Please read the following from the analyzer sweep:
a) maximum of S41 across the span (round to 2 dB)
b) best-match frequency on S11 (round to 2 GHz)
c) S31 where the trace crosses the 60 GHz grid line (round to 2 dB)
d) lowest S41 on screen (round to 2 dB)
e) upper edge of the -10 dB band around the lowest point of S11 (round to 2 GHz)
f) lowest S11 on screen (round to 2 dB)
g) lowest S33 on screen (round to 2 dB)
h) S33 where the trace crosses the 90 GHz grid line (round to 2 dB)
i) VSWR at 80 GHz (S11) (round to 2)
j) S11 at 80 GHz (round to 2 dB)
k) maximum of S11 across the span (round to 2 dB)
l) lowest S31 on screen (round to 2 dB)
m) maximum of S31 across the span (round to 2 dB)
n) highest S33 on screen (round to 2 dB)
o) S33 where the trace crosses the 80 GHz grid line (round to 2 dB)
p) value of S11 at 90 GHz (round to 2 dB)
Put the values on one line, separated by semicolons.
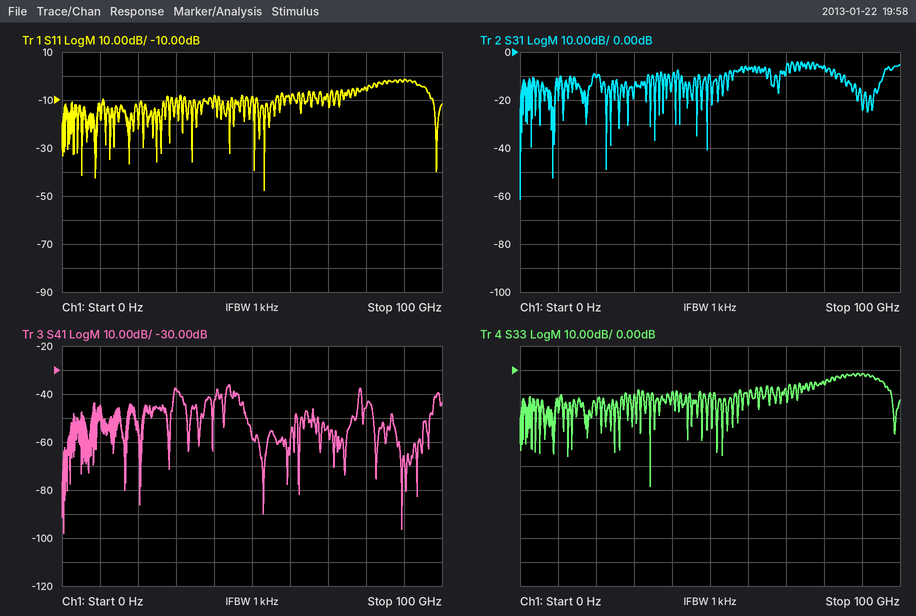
-36 dB; 54 GHz; -8 dB; -98 dB; 56 GHz; -48 dB; -48 dB; -2 dB; 4; -6 dB; -2 dB; -62 dB; -4 dB; -2 dB; -6 dB; -2 dB
